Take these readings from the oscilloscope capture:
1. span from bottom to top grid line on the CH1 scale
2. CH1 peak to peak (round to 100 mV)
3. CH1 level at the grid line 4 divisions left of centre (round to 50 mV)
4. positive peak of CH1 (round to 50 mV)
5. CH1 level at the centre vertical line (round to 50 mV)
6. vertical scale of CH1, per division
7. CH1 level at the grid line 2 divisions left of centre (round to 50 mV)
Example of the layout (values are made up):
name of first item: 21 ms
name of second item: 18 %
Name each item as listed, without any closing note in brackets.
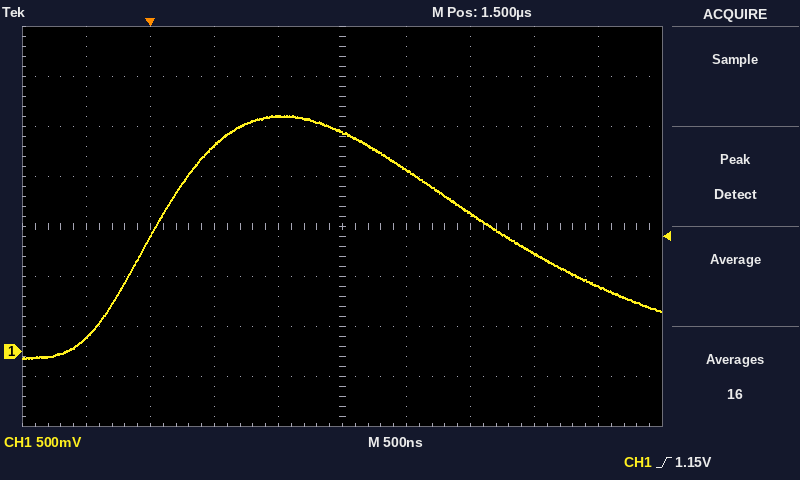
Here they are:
span from bottom to top grid line on the CH1 scale: 4 V
CH1 peak to peak: 2.40 V
CH1 level at the grid line 4 divisions left of centre: 150 mV
positive peak of CH1: 2.35 V
CH1 level at the centre vertical line: 2.20 V
vertical scale of CH1, per division: 500 mV
CH1 level at the grid line 2 divisions left of centre: 2.05 V
